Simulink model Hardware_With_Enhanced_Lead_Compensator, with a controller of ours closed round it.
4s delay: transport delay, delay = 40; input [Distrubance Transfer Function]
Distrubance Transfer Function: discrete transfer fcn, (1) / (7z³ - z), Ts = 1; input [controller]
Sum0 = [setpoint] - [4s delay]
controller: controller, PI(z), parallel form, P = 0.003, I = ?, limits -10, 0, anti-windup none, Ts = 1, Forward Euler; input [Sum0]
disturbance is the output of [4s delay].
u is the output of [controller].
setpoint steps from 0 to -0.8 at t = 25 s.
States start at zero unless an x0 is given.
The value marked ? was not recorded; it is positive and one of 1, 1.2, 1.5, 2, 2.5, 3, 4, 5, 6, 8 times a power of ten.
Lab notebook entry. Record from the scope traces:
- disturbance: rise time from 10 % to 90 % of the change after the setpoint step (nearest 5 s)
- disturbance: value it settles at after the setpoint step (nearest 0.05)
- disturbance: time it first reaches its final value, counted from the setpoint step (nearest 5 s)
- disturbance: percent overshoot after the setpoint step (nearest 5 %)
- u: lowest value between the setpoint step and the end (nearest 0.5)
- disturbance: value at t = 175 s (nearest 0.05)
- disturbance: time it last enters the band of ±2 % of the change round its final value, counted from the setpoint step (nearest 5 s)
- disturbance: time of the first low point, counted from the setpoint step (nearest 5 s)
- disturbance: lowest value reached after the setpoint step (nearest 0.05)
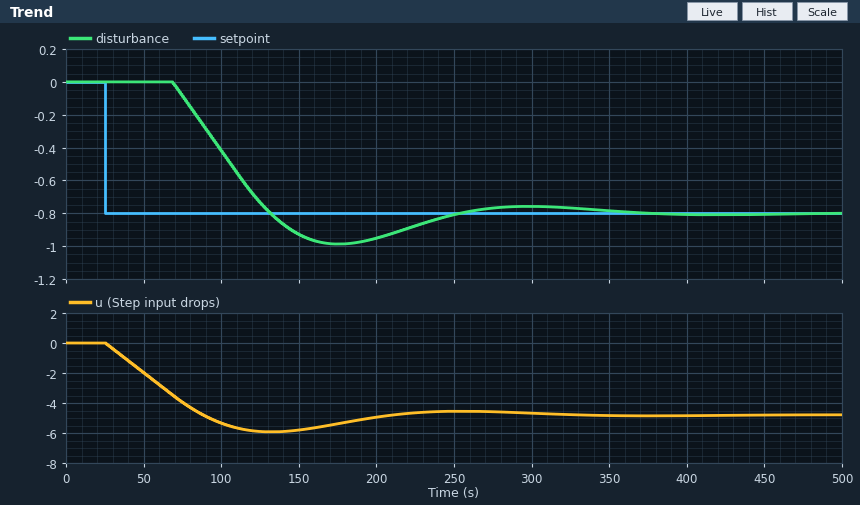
50 s
-0.80
105 s
25 %
-6.0
-1.00
325 s
150 s
-1.00
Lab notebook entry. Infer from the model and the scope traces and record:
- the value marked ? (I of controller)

0.1
